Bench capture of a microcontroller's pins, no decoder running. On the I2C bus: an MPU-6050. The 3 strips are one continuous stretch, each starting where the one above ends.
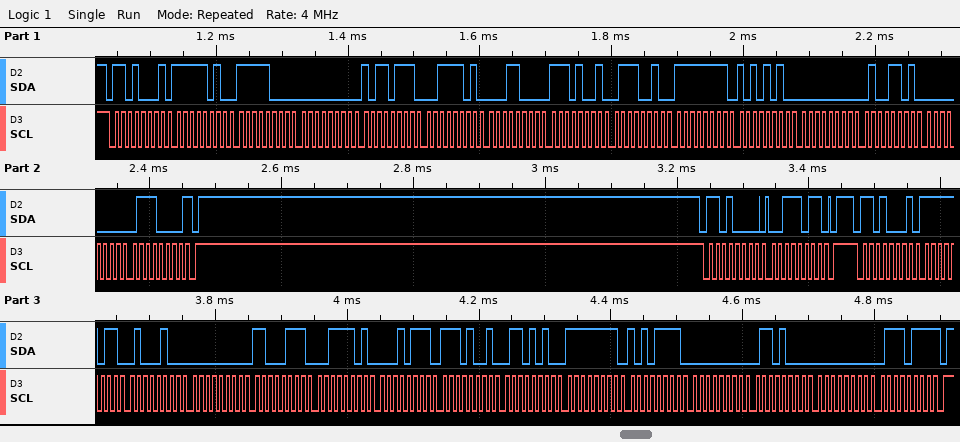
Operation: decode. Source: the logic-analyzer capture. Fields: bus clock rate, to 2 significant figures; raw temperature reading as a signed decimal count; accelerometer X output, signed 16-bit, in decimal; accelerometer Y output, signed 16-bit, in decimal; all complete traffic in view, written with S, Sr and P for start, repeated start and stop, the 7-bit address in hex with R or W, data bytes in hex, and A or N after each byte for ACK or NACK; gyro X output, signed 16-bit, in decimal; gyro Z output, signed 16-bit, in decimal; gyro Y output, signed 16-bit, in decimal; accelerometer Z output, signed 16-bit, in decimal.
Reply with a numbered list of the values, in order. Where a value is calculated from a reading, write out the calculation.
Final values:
1. 100 kHz
2. 0xE96A = -5782
3. 0xFB44 = -1212
4. 0x00C7 = 199
5. S 68R A FA A F8 A 00 A B7 A 3D A 18 A E9 A 72 A FF A AA A 00 A 4D A 00 A 70 N P S 68W A 3B A P S 68R A FB A 44 A 00 A C7 A 3D A 17 A E9 A 6A A FF A AF A 00 A 68 A 00 A 77 N P
6. 0xFFAF = -81
7. 0x0077 = 119
8. 0x0068 = 104
9. 0x3D17 = 15639
